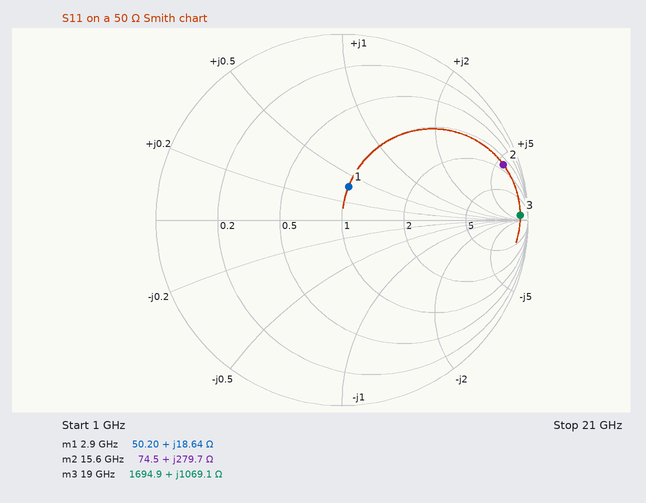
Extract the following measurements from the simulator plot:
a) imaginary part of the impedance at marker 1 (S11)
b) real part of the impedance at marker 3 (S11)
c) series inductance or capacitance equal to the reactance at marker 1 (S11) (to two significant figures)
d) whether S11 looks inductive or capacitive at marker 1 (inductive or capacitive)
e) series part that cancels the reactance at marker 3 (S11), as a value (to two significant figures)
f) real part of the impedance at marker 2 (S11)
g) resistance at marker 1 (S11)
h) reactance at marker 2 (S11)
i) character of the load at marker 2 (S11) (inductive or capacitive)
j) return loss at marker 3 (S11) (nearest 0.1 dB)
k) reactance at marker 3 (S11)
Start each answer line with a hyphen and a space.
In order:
- +18.64 Ω
- 1694.9 Ω
- 1.0 nH
- inductive
- 7.8 fF
- 74.5 Ω
- 50.20 Ω
- +279.7 Ω
- inductive
- 0.4 dB
- +1069.1 Ω
